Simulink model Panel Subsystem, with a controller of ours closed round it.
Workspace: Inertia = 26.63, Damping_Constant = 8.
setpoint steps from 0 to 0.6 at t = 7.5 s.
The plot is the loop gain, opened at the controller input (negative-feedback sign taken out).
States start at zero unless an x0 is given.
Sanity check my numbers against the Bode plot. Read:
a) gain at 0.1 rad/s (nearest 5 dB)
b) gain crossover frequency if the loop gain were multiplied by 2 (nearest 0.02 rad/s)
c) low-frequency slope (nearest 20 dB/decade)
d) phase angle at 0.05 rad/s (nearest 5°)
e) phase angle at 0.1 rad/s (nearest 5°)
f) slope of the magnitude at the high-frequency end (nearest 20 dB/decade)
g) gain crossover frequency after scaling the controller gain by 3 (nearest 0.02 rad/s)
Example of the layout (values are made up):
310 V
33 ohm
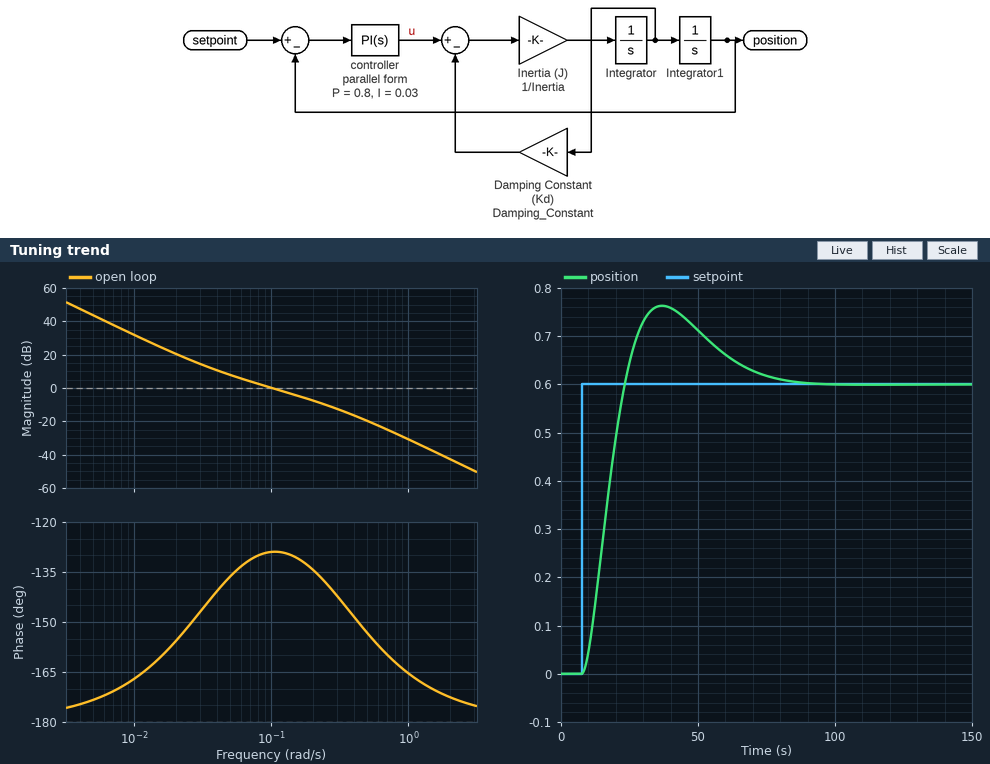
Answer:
0 dB
0.18 rad/s
-40 dB/decade
-135°
-130°
-40 dB/decade
0.24 rad/s
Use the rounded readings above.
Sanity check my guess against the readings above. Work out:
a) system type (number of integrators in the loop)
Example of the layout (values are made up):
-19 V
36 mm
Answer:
2
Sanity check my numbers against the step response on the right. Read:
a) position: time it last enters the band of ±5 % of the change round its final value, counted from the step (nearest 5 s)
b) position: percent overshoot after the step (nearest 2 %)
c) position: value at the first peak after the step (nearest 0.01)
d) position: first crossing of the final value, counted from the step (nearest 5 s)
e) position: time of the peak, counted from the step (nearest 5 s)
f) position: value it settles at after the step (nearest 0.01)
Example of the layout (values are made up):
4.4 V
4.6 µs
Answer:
60 s
28 %
0.76
15 s
30 s
0.60
